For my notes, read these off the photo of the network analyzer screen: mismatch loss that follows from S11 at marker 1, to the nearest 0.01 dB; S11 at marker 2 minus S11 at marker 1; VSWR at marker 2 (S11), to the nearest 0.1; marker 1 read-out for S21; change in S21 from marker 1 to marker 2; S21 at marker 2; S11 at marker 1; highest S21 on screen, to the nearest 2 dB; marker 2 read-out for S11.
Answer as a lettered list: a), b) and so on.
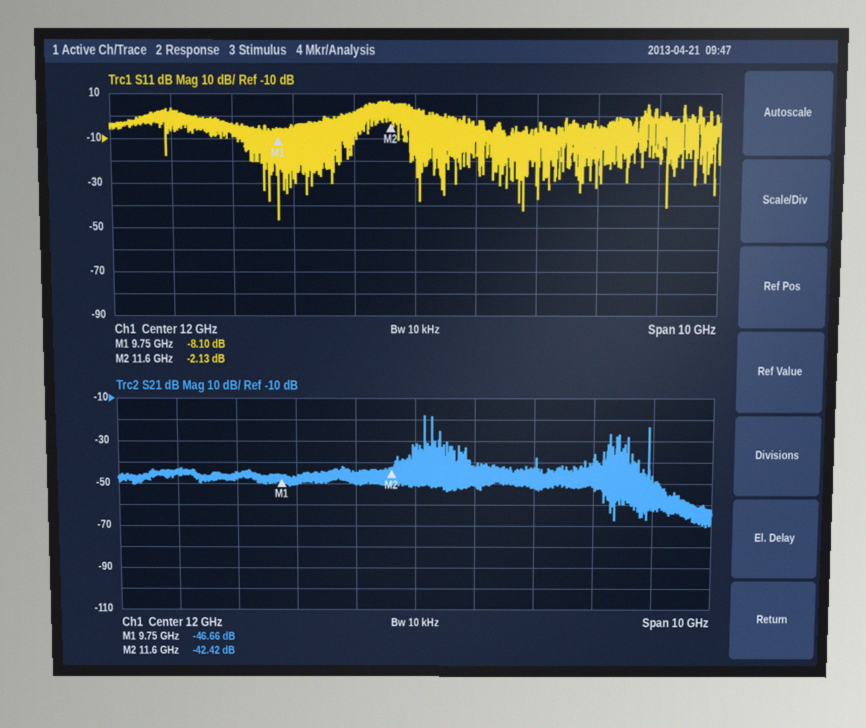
a) 0.73 dB
b) 5.97 dB
c) 8.2
d) -46.66 dB
e) 4.24 dB
f) -42.42 dB
g) -8.10 dB
h) -18 dB
i) -2.13 dB
